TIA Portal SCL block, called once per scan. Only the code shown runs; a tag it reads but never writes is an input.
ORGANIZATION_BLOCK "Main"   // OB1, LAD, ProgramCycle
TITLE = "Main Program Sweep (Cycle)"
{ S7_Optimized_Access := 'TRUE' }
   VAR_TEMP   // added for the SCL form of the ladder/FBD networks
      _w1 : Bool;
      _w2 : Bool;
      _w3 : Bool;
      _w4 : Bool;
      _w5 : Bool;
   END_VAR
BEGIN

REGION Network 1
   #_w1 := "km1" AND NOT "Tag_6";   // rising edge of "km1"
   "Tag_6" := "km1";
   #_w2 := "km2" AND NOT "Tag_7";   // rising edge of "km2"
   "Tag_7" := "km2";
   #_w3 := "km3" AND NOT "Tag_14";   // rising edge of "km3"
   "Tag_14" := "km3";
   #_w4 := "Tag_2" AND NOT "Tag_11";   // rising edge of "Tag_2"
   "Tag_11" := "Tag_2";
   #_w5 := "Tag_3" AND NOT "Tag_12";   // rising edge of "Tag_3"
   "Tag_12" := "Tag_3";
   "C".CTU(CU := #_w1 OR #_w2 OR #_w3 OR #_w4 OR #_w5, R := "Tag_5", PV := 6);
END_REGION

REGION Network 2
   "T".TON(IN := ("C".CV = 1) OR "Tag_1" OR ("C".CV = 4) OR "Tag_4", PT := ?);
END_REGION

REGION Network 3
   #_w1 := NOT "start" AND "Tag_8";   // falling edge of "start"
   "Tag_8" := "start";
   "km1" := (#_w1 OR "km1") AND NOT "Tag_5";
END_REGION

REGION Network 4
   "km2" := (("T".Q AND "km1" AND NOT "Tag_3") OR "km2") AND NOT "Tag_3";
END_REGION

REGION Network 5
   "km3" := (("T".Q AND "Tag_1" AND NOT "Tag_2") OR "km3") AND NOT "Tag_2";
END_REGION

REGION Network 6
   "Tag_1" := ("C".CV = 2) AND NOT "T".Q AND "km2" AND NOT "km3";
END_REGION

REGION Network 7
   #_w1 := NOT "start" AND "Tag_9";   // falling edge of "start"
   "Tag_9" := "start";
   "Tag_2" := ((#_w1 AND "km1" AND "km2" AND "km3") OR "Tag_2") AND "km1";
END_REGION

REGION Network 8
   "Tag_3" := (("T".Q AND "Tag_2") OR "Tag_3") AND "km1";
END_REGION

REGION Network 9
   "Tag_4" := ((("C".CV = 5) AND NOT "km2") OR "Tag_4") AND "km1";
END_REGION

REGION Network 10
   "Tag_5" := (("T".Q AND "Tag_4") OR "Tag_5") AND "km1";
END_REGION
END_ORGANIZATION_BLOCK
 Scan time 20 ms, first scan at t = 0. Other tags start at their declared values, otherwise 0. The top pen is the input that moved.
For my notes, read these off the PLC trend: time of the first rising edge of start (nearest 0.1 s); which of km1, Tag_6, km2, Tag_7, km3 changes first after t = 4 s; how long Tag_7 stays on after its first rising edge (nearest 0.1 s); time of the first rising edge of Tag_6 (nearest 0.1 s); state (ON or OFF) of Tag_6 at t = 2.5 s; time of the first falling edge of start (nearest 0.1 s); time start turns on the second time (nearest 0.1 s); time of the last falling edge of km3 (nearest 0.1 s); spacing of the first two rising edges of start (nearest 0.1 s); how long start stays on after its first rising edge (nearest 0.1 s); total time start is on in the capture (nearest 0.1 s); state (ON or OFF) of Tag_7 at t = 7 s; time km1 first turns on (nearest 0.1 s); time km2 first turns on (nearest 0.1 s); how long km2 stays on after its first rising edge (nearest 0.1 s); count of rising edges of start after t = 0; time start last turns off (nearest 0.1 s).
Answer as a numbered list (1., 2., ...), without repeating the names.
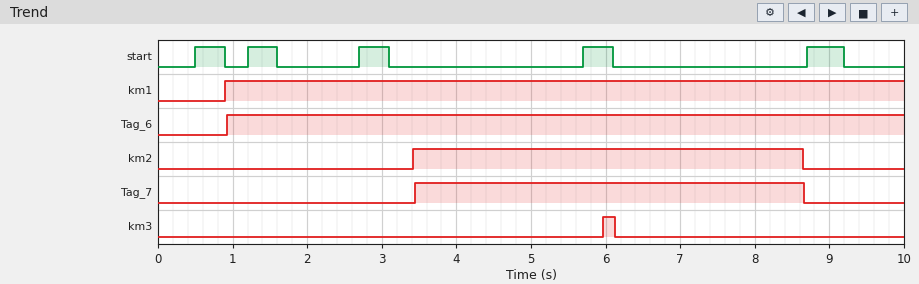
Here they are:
1. 0.5 s
2. km3
3. 5.2 s
4. 0.9 s
5. ON
6. 0.9 s
7. 1.2 s
8. 6.1 s
9. 0.7 s
10. 0.4 s
11. 2.1 s
12. ON
13. 0.9 s
14. 3.4 s
15. 5.2 s
16. 5
17. 9.2 s
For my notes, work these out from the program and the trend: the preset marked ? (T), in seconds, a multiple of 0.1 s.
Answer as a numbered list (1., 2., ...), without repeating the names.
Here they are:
1. 2.5 s
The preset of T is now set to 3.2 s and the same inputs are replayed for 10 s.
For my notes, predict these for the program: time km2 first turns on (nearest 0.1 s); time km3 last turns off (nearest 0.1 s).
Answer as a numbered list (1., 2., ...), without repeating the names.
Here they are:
1. 4.1 s
2. 9.2 s
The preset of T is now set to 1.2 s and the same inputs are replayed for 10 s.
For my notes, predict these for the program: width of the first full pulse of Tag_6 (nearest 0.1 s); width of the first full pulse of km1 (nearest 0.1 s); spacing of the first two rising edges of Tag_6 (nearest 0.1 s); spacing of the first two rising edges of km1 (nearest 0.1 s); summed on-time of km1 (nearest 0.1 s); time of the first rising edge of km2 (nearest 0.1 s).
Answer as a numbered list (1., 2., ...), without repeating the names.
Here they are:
1. 7.7 s
2. 7.7 s
3. 8.3 s
4. 8.3 s
5. 8.5 s
6. 2.1 s
